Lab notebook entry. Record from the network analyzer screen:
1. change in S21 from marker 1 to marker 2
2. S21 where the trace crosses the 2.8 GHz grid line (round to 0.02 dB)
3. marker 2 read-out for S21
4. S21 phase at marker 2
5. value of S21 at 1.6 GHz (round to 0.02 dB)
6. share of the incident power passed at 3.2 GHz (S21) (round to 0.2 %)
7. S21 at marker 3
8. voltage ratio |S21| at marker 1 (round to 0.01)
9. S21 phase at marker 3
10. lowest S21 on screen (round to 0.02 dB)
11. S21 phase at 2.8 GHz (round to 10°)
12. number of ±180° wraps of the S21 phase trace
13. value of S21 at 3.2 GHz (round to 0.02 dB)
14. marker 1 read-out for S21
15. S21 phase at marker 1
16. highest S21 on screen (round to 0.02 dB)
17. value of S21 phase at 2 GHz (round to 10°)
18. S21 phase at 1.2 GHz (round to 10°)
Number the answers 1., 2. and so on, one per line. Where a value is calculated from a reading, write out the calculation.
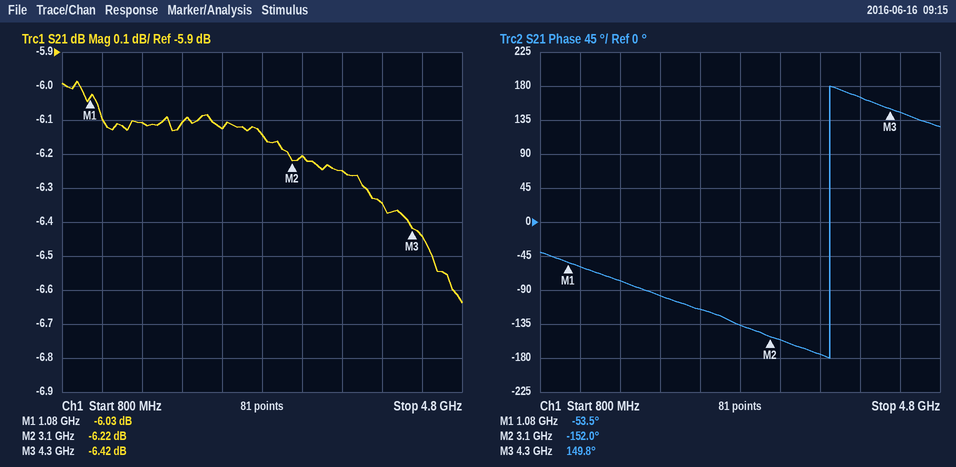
1. -6.22 − (-6.03) = -0.19 dB
2. -6.14 dB
3. -6.22 dB
4. -152.0°
5. -6.10 dB
6. 10^(-6.2/10) ≈ 24.0 %
7. -6.42 dB
8. 10^(-6.03/20) ≈ 0.50
9. 149.8°
10. -6.64 dB
11. -140°
12. 1
13. -6.20 dB
14. -6.03 dB
15. -53.5°
16. -5.98 dB
17. -100°
18. -60°
